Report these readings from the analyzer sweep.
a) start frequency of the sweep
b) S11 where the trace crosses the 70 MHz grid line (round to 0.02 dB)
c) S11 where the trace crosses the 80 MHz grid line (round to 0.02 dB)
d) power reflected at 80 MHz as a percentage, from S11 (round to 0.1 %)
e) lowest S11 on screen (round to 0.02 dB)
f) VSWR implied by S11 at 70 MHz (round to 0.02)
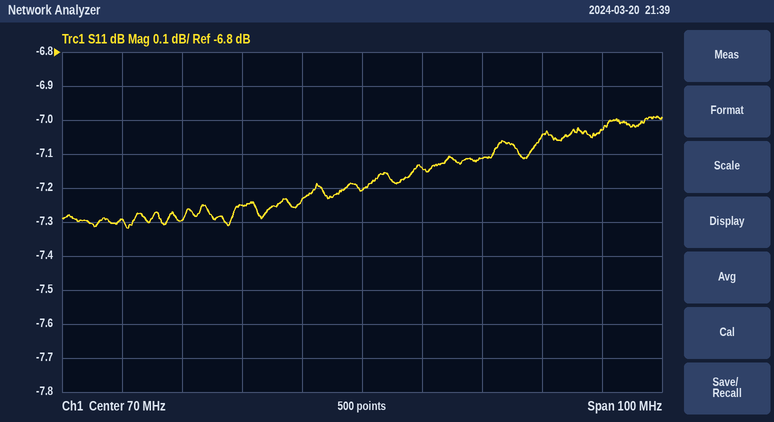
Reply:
20 MHz
-7.20 dB
-7.14 dB
19.3 %
-7.32 dB
2.54
